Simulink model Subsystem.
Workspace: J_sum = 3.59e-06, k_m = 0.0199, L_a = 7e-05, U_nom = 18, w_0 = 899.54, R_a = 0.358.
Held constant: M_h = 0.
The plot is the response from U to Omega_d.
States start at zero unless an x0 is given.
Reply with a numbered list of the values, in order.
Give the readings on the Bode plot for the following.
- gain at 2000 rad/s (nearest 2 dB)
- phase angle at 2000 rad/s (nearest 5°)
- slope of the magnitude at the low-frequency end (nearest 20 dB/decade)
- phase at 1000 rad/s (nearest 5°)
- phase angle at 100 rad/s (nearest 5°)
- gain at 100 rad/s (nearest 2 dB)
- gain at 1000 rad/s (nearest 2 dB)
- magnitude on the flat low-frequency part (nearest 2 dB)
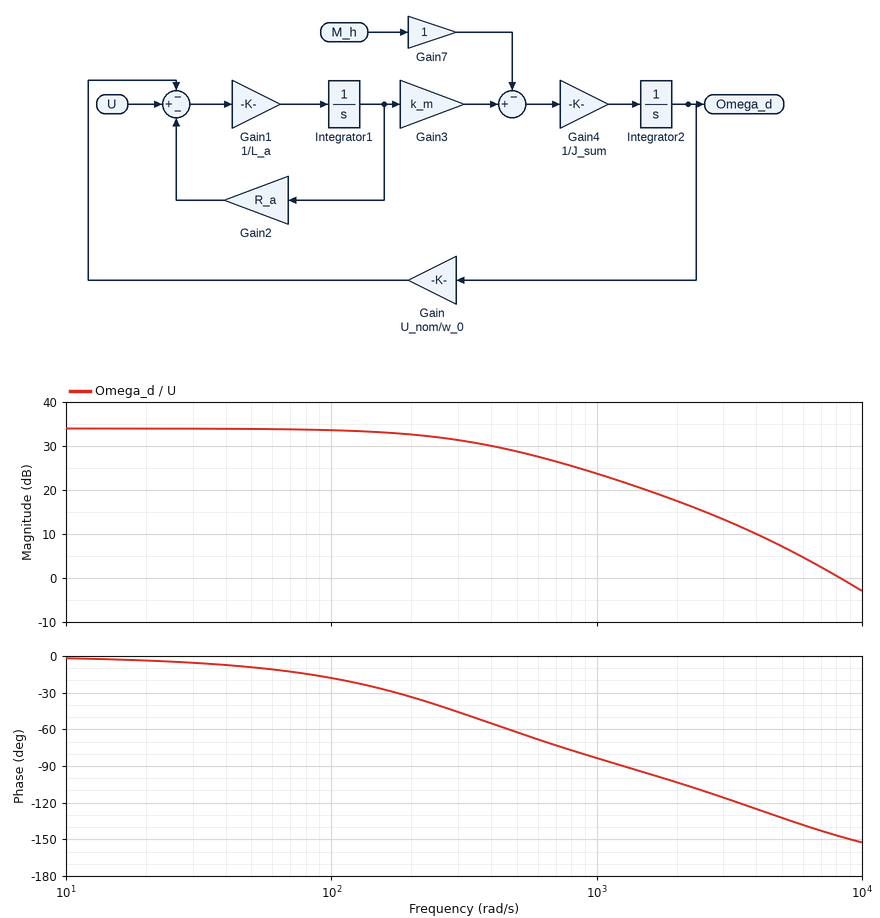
1. 18 dB
2. -105°
3. 0 dB/decade
4. -85°
5. -20°
6. 34 dB
7. 24 dB
8. 34 dB
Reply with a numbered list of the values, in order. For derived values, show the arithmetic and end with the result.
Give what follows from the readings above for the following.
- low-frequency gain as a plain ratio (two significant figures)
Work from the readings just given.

1. 10^(34 / 20) = 50
